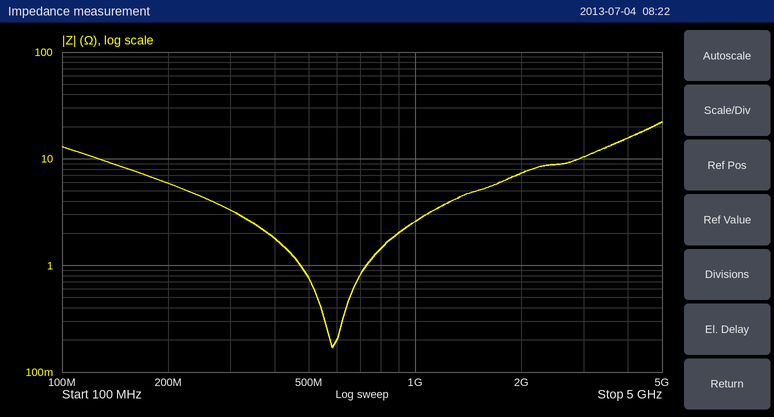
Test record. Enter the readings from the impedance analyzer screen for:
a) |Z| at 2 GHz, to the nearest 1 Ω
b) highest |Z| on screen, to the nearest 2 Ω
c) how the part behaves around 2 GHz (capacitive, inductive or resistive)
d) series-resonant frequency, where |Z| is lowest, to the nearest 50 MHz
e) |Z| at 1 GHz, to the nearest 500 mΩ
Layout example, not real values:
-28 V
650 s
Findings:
7 Ω
22 Ω
inductive
600 MHz
2.5 Ω
